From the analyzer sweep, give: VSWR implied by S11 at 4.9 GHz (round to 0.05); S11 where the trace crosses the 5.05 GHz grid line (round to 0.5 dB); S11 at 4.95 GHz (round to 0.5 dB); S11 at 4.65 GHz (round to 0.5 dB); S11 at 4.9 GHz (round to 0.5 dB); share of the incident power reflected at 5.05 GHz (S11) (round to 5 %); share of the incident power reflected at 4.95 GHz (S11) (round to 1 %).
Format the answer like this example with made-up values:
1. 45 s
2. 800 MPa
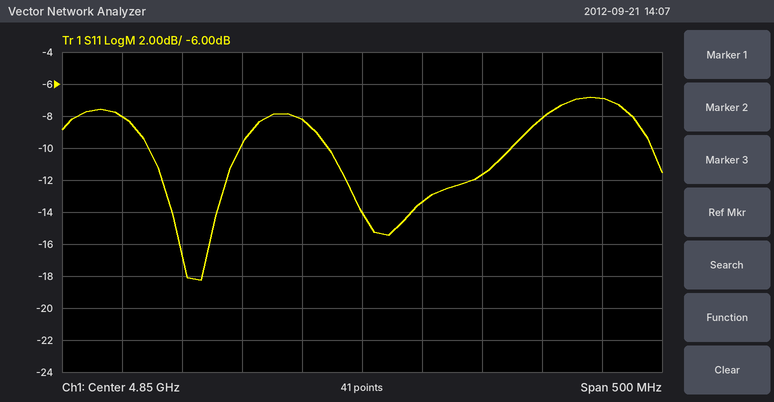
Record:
1. 1.55
2. -7.0 dB
3. -11.5 dB
4. -8.0 dB
5. -13.5 dB
6. 20 %
7. 7 %
